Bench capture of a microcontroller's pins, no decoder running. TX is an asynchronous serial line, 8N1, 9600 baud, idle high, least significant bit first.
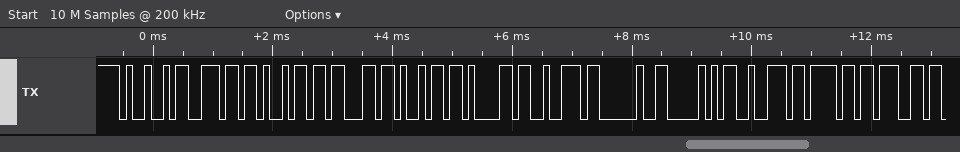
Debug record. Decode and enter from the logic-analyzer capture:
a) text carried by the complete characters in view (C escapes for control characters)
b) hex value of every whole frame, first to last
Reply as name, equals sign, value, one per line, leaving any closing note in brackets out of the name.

text carried by the complete characters in view = "Iniciar Prog"
hex value of every whole frame, first to last = 0x49 0x6E 0x69 0x63 0x69 0x61 0x72 0x20 0x50 0x72 0x6F 0x67
